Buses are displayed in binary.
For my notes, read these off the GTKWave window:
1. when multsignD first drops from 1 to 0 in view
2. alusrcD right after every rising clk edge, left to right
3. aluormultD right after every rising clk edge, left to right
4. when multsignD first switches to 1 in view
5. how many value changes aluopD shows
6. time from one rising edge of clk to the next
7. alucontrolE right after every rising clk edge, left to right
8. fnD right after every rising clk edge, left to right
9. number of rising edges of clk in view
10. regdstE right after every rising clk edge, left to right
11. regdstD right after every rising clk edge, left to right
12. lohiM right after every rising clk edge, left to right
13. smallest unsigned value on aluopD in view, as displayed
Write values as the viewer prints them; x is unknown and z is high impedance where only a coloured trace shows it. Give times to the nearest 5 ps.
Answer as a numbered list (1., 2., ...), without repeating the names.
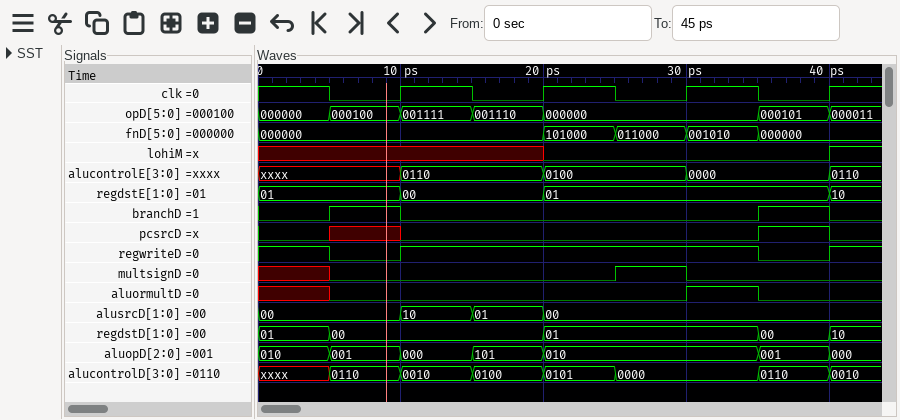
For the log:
1. 30 ps
2. 10, 00, 00, 00
3. 0 0 1 0
4. 25 ps
5. 6
6. 10 ps
7. 0110, 0100, 0000, 0110
8. 000000, 101000, 001010, 000000
9. 4
10. 00, 01, 01, 10
11. 00, 01, 01, 10
12. x 0 0 1
13. 000
